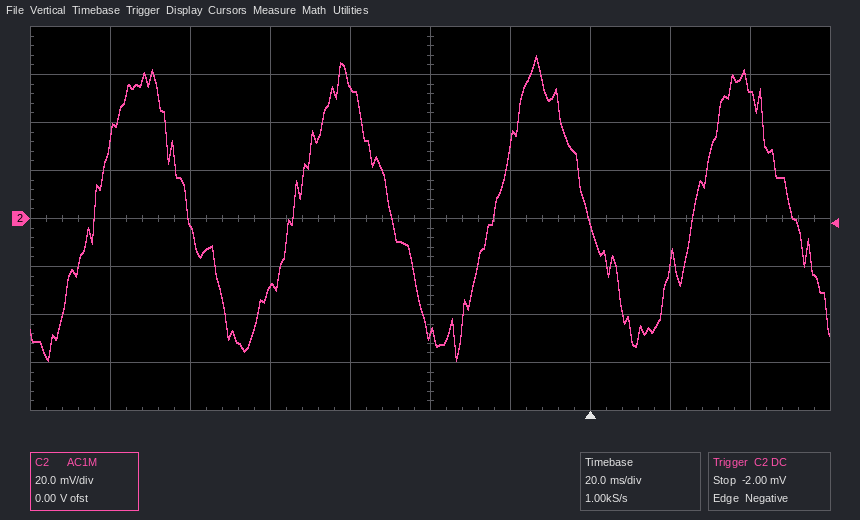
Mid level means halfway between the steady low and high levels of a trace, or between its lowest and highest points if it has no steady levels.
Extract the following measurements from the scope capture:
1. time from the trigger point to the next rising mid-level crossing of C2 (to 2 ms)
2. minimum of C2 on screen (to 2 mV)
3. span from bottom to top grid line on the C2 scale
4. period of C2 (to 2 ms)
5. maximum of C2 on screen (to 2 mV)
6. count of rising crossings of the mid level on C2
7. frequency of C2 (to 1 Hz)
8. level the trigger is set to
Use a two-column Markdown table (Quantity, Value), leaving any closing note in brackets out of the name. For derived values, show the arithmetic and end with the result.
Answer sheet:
| Quantity | Value |
|---|---|
| time from the trigger point to the next rising mid-level crossing of C2 | 26 ms |
| minimum of C2 on screen | -60 mV |
| span from bottom to top grid line on the C2 scale | 160 mV |
| period of C2 | 50 ms |
| maximum of C2 on screen | 68 mV |
| count of rising crossings of the mid level on C2 | 4 |
| frequency of C2 | 1 / 50 ms ≈ 20 Hz |
| level the trigger is set to | -2.00 mV |
